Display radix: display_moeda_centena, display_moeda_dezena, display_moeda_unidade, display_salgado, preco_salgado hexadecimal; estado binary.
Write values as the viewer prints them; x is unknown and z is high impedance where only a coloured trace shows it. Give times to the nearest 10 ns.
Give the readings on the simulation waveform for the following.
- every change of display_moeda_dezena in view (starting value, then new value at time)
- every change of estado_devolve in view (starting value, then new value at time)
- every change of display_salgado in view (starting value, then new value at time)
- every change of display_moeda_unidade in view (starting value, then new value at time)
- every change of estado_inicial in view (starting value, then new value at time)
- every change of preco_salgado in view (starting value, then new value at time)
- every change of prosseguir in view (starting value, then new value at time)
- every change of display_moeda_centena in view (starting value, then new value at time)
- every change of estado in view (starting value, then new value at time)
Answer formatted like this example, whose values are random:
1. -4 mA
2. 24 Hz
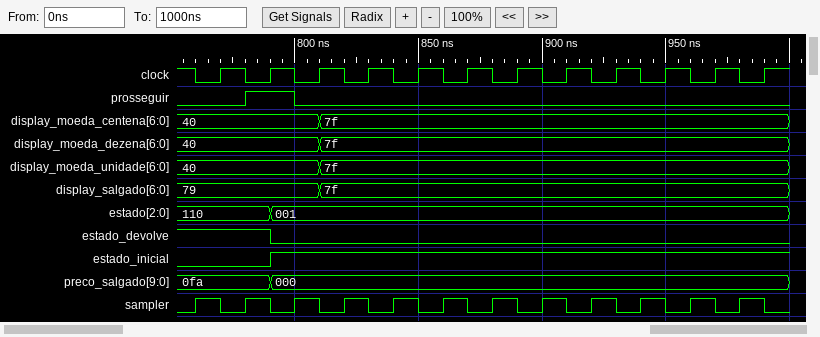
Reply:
1. 40, 7f at 810 ns
2. 1, 0 at 790 ns
3. 79, 7f at 810 ns
4. 40, 7f at 810 ns
5. 0, 1 at 790 ns
6. 0fa, 000 at 790 ns
7. 0, 1 at 780 ns, 0 at 800 ns
8. 40, 7f at 810 ns
9. 110, 001 at 790 ns
